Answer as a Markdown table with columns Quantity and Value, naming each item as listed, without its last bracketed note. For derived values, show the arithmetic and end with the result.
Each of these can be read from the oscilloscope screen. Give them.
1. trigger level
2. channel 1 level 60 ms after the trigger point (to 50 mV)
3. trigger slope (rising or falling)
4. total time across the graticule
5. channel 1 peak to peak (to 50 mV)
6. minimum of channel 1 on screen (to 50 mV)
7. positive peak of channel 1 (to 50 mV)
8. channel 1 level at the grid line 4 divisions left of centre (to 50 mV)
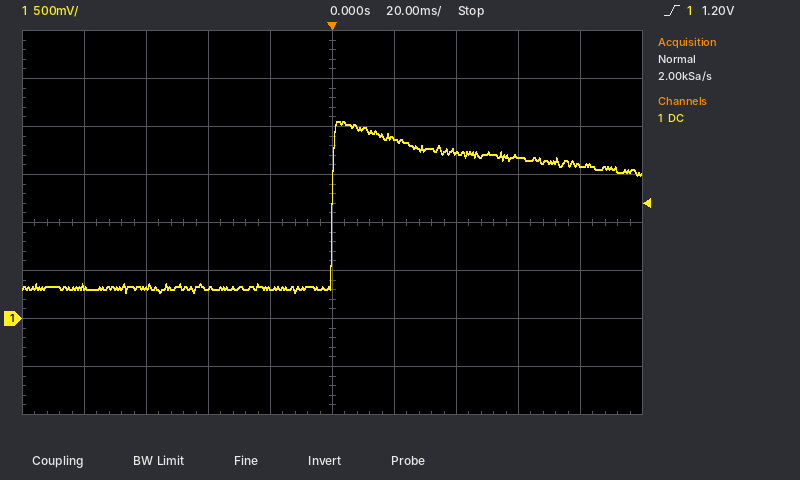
| Quantity | Value |
|---|---|
| trigger level | 1.20 V |
| channel 1 level 60 ms after the trigger point | 1.70 V |
| trigger slope | rising |
| total time across the graticule | 200 ms |
| channel 1 peak to peak | 2.05 V − (250 mV) = 1.80 V |
| minimum of channel 1 on screen | 250 mV |
| positive peak of channel 1 | 2.05 V |
| channel 1 level at the grid line 4 divisions left of centre | 350 mV |
